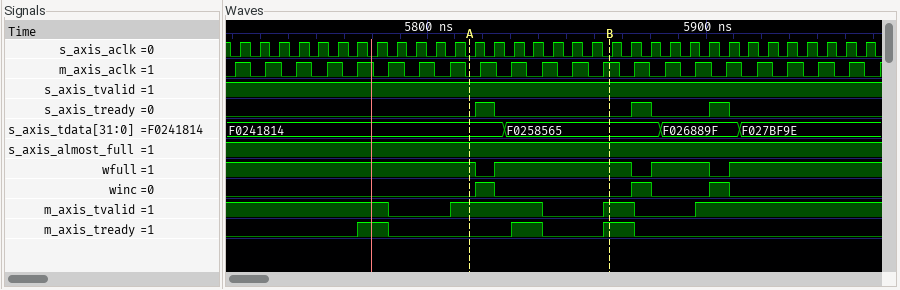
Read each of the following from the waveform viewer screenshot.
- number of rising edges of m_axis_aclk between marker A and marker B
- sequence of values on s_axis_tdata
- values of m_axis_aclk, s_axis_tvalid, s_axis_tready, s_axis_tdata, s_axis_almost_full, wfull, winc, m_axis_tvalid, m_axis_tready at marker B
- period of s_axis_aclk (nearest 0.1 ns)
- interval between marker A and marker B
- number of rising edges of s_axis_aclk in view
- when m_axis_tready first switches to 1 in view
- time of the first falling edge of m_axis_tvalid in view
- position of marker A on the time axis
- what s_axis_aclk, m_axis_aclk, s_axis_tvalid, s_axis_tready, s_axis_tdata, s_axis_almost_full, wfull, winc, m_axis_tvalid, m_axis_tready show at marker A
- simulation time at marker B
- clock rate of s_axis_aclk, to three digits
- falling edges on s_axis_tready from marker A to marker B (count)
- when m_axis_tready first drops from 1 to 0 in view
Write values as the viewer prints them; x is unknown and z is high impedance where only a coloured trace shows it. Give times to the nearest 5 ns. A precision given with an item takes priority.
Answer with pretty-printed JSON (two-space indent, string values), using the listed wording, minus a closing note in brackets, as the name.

{
  "number of rising edges of m_axis_aclk between marker A and marker B": "5",
  "sequence of values on s_axis_tdata": "F0241814, F0258565, F026889F, F027BF9E",
  "values of m_axis_aclk, s_axis_tvalid, s_axis_tready, s_axis_tdata, s_axis_almost_full, wfull, winc, m_axis_tvalid, m_axis_tready at marker B": "m_axis_aclk=1, s_axis_tvalid=1, s_axis_tready=0, s_axis_tdata=F0258565, s_axis_almost_full=1, wfull=1, winc=0, m_axis_tvalid=1, m_axis_tready=1",
  "period of s_axis_aclk": "7 ns",
  "interval between marker A and marker B": "50 ns",
  "number of rising edges of s_axis_aclk in view": "33",
  "when m_axis_tready first switches to 1 in view": "5775 ns",
  "time of the first falling edge of m_axis_tvalid in view": "5785 ns",
  "position of marker A on the time axis": "5815 ns",
  "what s_axis_aclk, m_axis_aclk, s_axis_tvalid, s_axis_tready, s_axis_tdata, s_axis_almost_full, wfull, winc, m_axis_tvalid, m_axis_tready show at marker A": "s_axis_aclk=0, m_axis_aclk=0, s_axis_tvalid=1, s_axis_tready=0, s_axis_tdata=F0241814, s_axis_almost_full=1, wfull=1, winc=0, m_axis_tvalid=1, m_axis_tready=0",
  "simulation time at marker B": "5865 ns",
  "clock rate of s_axis_aclk, to three digits": "143 MHz",
  "falling edges on s_axis_tready from marker A to marker B": "1",
  "when m_axis_tready first drops from 1 to 0 in view": "5785 ns"
}
